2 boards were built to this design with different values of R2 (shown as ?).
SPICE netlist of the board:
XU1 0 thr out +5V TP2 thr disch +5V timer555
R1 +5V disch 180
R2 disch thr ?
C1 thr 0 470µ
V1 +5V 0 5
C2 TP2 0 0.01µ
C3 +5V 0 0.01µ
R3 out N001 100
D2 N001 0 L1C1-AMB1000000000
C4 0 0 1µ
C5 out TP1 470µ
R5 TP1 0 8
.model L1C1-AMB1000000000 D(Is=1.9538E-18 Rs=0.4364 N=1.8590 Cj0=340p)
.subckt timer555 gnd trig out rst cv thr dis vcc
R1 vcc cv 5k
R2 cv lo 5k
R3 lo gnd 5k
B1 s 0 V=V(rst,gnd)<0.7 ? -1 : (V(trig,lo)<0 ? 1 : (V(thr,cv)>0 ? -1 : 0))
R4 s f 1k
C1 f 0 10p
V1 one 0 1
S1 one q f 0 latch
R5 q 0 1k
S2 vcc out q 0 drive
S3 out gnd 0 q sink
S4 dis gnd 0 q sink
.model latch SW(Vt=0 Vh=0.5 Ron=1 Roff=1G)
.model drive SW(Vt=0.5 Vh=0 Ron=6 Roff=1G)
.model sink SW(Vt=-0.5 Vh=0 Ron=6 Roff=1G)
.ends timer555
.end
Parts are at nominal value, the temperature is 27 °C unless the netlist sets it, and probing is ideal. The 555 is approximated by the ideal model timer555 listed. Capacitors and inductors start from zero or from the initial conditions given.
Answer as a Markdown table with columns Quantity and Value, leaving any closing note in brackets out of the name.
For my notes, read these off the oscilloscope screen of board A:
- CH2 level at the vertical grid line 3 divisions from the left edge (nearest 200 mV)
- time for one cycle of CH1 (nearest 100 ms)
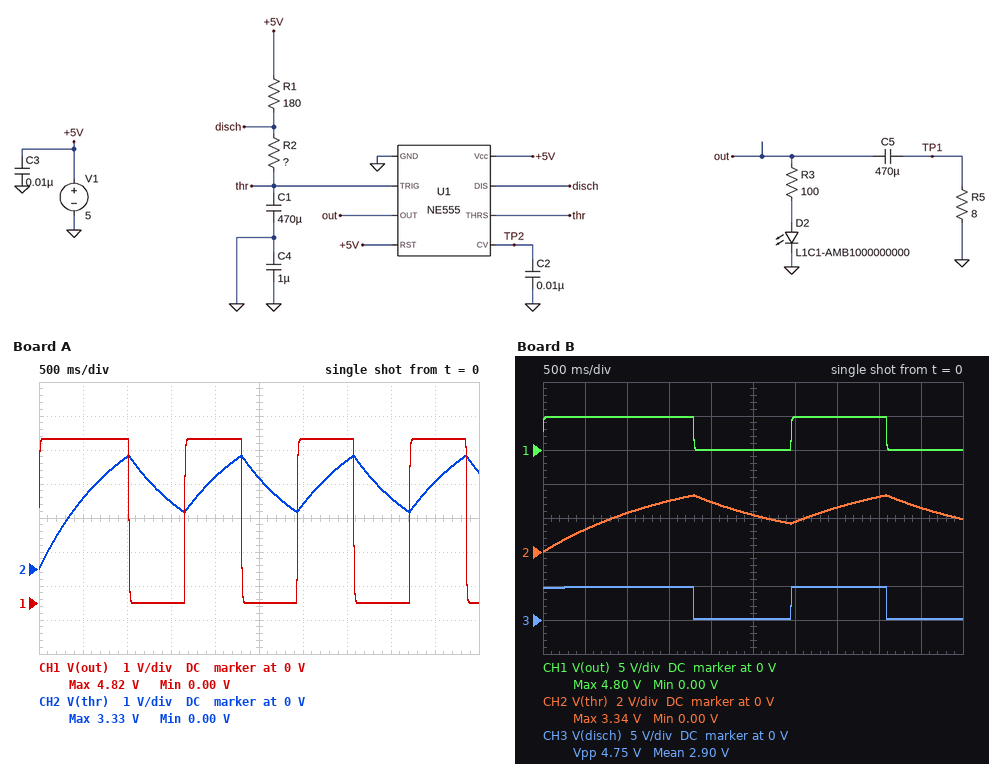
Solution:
| Quantity | Value |
|---|---|
| CH2 level at the vertical grid line 3 divisions from the left edge | 2.0 V |
| time for one cycle of CH1 | 1.3 s |
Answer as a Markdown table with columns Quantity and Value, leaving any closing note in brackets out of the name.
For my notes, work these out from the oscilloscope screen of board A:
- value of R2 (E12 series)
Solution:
| Quantity | Value |
|---|---|
| value of R2 | 1.8 kΩ |
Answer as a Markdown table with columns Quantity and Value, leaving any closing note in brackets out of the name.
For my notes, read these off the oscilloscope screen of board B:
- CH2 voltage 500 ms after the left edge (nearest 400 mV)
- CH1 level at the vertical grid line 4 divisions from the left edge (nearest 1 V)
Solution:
| Quantity | Value |
|---|---|
| CH2 voltage 500 ms after the left edge | 1.2 V |
| CH1 level at the vertical grid line 4 divisions from the left edge | 0 V |
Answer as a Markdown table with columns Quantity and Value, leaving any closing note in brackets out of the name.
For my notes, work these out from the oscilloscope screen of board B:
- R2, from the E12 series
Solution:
| Quantity | Value |
|---|---|
| R2, from the E12 series | 3.3 kΩ |
